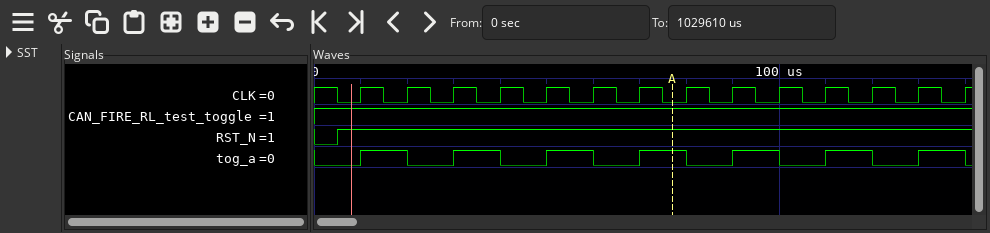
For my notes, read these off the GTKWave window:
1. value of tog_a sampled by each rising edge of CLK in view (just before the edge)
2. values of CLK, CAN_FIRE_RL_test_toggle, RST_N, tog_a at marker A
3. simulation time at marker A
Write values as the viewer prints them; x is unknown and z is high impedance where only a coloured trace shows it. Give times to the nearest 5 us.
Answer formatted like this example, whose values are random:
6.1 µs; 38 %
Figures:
0 1 0 1 0 1 0 1 0 1 0 1 0 1; CLK=0, CAN_FIRE_RL_test_toggle=1, RST_N=1, tog_a=1; 75 us
